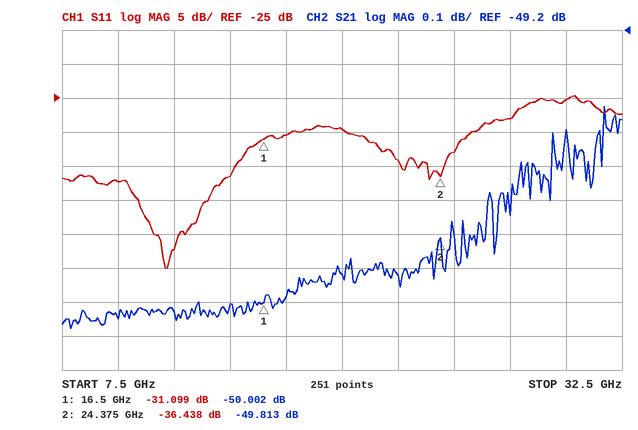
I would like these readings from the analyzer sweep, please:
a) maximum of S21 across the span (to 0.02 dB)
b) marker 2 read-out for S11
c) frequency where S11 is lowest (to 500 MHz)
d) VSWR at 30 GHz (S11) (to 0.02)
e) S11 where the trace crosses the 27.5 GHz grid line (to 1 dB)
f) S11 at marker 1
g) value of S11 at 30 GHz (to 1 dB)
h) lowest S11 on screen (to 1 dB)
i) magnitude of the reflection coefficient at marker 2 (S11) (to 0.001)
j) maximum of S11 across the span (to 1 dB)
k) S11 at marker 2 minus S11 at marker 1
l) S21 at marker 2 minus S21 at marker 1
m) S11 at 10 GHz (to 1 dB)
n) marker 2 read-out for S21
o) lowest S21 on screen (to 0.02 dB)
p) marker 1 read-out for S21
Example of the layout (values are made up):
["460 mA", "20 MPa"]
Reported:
["-49.42 dB", "-36.438 dB", "12.0 GHz", "1.12", "-28 dB", "-31.099 dB", "-25 dB", "-50 dB", "0.015", "-25 dB", "-5.339 dB", "0.189 dB", "-37 dB", "-49.813 dB", "-50.08 dB", "-50.002 dB"]
